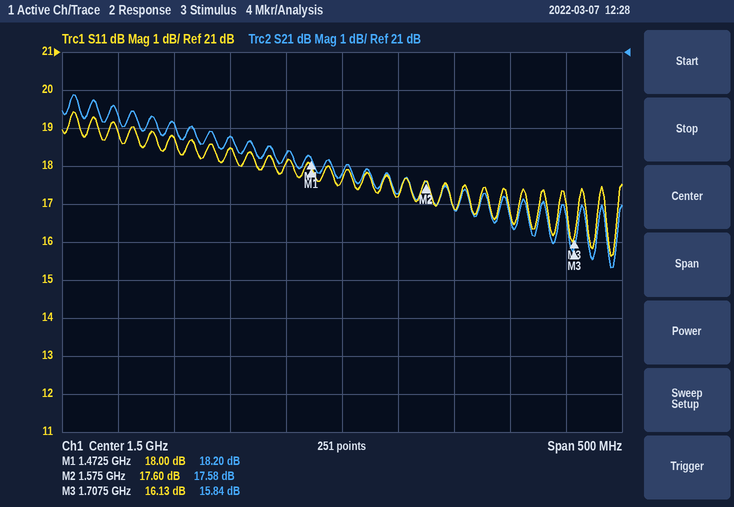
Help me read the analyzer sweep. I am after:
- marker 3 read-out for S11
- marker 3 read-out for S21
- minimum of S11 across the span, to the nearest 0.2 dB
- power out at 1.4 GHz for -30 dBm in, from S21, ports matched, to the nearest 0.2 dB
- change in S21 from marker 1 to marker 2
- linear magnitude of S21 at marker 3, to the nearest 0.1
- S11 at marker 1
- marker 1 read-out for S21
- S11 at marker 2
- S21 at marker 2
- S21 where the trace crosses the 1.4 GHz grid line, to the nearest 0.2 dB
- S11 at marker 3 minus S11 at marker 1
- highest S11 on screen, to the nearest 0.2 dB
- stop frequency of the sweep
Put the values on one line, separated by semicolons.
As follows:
16.13 dB; 15.84 dB; 15.6 dB; -11.2 dBm; -0.62 dB; 6.2; 18.00 dB; 18.20 dB; 17.60 dB; 17.58 dB; 18.8 dB; -1.87 dB; 19.4 dB; 1.75 GHz
